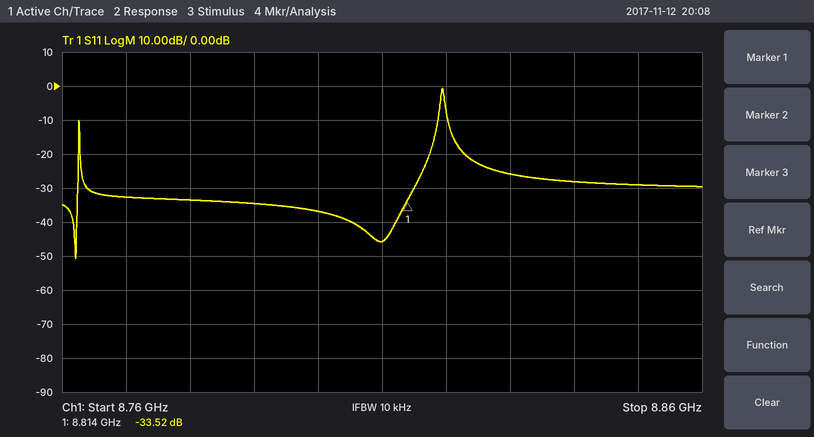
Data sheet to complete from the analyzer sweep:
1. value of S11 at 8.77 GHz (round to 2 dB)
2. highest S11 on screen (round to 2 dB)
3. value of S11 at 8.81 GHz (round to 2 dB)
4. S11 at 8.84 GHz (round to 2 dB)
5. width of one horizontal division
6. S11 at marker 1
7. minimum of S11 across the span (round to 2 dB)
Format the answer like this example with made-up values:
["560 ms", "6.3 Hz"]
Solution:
["-32 dB", "0 dB", "-46 dB", "-28 dB", "10 MHz", "-33.52 dB", "-50 dB"]
